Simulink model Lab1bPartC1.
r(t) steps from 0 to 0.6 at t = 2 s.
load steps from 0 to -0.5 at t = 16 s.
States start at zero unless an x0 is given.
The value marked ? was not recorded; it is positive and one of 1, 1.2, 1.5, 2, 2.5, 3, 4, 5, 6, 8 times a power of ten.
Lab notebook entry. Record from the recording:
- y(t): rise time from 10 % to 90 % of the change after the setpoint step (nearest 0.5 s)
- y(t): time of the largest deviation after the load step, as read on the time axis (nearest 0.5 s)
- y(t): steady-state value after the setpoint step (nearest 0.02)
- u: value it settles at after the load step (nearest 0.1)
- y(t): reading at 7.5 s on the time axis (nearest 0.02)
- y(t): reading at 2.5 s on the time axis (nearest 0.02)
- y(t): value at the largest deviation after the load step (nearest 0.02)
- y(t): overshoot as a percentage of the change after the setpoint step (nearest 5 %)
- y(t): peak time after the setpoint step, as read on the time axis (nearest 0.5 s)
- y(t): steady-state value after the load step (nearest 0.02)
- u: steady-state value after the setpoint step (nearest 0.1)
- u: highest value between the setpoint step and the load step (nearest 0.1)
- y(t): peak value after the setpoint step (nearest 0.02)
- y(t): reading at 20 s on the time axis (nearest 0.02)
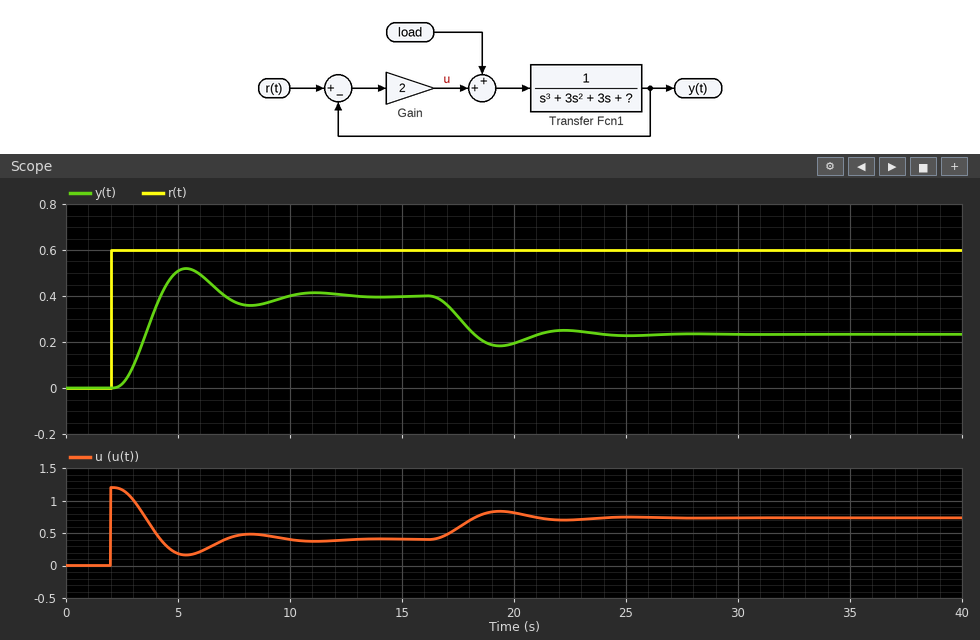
1.5 s
19.5 s
0.40
0.7
0.38
0.02
0.18
30 %
5.5 s
0.24
0.4
1.2
0.52
0.20
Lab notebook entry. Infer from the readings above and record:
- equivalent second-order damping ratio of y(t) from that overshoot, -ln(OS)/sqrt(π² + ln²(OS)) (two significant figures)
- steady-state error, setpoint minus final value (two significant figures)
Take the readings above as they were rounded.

0.36
0.20
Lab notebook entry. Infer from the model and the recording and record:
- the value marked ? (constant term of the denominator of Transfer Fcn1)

1
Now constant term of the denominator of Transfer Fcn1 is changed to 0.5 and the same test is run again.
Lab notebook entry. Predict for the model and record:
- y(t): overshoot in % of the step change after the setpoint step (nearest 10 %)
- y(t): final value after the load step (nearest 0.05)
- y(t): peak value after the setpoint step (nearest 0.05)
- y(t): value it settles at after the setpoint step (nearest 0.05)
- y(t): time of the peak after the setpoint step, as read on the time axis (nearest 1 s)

20 %
0.30
0.60
0.50
6 s
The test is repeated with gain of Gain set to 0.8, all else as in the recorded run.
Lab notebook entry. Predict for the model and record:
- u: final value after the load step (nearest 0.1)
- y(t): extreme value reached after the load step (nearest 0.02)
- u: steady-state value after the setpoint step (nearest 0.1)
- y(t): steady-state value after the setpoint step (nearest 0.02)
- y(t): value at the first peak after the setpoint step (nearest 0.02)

0.5
-0.04
0.3
0.26
0.30
